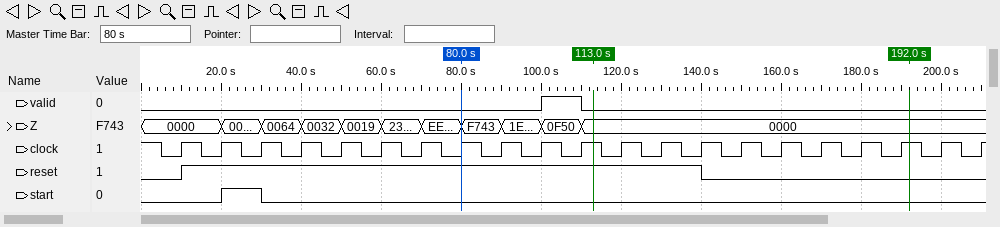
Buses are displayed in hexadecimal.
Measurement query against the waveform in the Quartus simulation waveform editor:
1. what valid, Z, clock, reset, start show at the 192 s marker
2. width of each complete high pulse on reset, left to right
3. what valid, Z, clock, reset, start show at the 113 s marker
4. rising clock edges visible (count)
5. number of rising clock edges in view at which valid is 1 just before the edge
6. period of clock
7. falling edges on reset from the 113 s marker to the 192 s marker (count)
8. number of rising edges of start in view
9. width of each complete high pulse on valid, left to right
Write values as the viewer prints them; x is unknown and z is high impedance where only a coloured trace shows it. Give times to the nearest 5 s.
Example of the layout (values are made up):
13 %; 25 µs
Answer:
valid=0, Z=0000, clock=1, reset=0, start=0; 130 s; valid=0, Z=0000, clock=1, reset=1, start=0; 21; 1; 10 s; 1; 1; 10 s
